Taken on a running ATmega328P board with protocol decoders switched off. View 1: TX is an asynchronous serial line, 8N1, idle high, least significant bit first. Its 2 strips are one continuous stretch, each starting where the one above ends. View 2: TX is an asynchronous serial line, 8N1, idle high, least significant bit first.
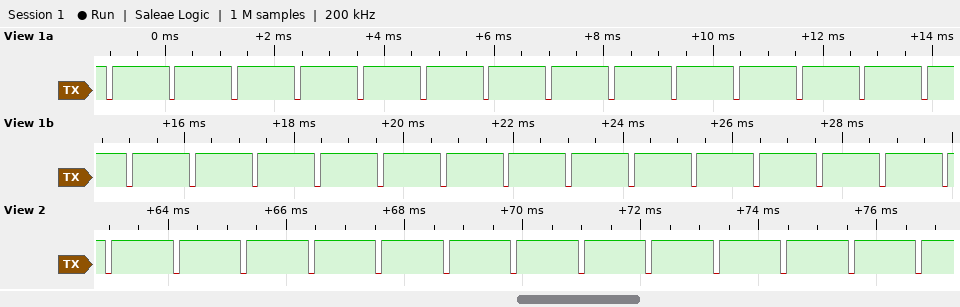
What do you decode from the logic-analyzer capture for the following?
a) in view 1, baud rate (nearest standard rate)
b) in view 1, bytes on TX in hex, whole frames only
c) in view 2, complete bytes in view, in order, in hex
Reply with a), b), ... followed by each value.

a) 9600 baud
b) FF FF FF FF FF FF FF FF FF FF FF FF FF FF FF FF FF FF FF FF FF FF FF FF FF FF FF
c) FF FF FF FF FF FF FF FF FF FF FF FF
